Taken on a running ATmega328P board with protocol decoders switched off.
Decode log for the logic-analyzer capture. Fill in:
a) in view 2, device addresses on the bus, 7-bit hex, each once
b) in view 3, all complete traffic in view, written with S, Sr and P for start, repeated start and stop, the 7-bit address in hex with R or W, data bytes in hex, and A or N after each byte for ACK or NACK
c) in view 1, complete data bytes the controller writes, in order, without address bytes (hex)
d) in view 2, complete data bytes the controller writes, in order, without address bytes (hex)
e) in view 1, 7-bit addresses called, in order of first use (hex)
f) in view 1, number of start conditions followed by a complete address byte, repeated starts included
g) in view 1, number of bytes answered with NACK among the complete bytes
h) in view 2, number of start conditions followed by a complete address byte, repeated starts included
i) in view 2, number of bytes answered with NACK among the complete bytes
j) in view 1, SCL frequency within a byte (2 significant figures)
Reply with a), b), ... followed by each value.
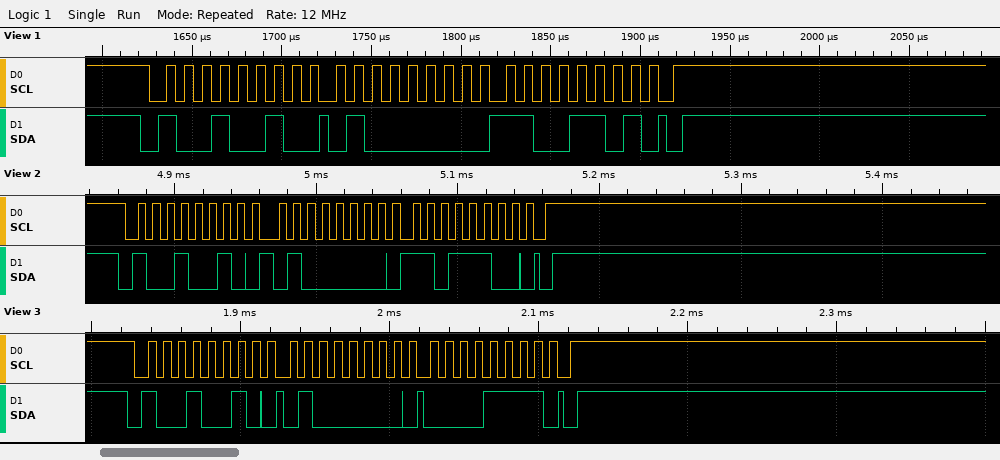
a) 0x49
b) S 49W A 40 A 0F A P
c) 40 CD
d) 40 DC
e) 0x49
f) 1
g) 0
h) 1
i) 0
j) 100 kHz
